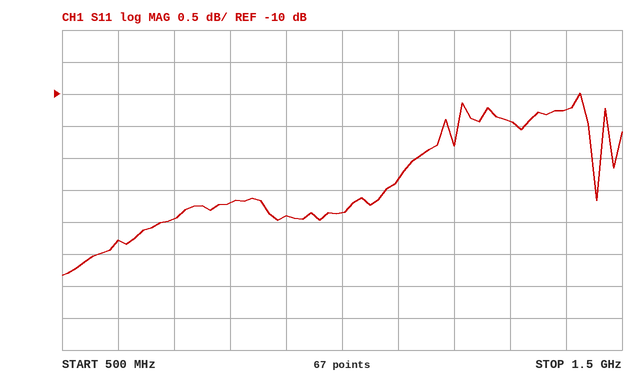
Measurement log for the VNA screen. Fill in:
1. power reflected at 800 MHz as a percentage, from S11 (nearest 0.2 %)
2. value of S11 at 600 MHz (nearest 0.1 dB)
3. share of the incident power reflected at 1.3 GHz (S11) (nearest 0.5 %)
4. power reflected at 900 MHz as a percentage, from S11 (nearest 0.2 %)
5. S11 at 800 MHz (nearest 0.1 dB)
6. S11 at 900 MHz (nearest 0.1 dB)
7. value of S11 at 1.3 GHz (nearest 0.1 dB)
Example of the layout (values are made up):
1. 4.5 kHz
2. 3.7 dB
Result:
1. 6.8 %
2. -12.3 dB
3. 9.0 %
4. 6.4 %
5. -11.7 dB
6. -11.9 dB
7. -10.4 dB
